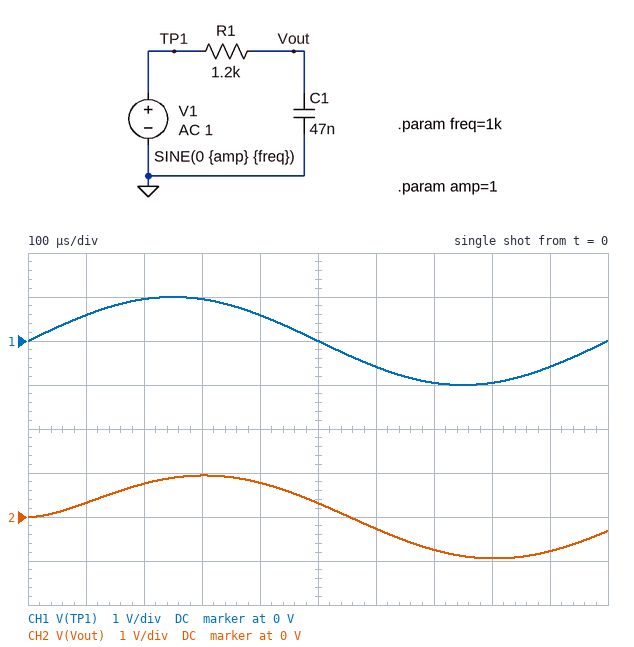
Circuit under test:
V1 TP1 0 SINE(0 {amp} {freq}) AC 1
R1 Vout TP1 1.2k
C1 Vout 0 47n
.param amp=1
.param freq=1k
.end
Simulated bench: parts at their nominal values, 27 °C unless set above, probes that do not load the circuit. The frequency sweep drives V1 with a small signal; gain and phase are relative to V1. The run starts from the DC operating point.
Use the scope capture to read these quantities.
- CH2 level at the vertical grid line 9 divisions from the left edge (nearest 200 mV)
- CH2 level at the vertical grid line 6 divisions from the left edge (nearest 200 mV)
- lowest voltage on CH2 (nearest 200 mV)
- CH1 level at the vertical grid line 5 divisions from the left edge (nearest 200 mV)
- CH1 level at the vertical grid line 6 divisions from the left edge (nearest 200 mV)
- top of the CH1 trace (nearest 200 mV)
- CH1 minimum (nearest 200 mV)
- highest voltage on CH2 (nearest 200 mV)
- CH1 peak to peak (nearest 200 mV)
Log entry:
-800 mV
-200 mV
-1.0 V
0 V
-600 mV
1.0 V
-1.0 V
1.0 V
2.0 V
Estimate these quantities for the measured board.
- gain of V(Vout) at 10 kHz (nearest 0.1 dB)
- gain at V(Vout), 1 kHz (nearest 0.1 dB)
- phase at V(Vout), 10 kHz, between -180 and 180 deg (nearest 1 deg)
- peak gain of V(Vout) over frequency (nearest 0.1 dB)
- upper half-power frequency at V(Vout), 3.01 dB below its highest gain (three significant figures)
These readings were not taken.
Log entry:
-11.3 dB
-0.5 dB
-74 deg
0 dB
2.82 kHz
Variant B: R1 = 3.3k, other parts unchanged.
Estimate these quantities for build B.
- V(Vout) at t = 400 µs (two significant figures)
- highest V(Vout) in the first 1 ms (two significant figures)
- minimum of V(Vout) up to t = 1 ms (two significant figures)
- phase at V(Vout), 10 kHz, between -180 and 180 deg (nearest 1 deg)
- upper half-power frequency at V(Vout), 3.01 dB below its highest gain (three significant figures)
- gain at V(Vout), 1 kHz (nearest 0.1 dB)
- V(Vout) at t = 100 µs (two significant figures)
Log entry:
740 mV
760 mV
-710 mV
-84 deg
1.03 kHz
-2.9 dB
160 mV
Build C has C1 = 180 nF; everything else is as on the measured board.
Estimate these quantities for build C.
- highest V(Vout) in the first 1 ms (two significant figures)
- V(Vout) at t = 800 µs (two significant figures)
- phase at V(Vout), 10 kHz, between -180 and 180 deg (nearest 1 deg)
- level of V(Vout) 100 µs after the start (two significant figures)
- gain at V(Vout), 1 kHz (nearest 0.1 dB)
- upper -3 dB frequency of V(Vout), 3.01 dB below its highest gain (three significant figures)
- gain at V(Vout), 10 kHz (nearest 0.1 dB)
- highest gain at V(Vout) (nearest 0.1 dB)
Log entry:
670 mV
-470 mV
-86 deg
120 mV
-4.5 dB
737 Hz
-22.7 dB
0 dB
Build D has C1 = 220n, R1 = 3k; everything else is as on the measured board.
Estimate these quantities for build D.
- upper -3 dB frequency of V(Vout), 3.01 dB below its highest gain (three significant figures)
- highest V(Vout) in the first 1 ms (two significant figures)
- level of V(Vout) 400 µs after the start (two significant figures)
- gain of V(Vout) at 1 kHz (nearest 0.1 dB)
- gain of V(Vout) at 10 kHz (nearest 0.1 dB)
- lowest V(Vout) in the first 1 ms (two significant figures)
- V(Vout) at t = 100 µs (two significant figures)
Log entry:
241 Hz
350 mV
340 mV
-12.6 dB
-32.4 dB
-180 mV
44 mV
